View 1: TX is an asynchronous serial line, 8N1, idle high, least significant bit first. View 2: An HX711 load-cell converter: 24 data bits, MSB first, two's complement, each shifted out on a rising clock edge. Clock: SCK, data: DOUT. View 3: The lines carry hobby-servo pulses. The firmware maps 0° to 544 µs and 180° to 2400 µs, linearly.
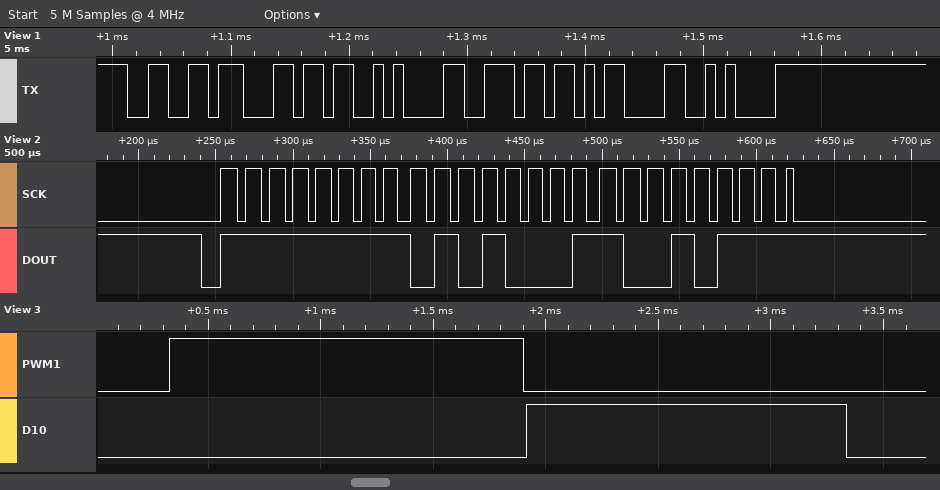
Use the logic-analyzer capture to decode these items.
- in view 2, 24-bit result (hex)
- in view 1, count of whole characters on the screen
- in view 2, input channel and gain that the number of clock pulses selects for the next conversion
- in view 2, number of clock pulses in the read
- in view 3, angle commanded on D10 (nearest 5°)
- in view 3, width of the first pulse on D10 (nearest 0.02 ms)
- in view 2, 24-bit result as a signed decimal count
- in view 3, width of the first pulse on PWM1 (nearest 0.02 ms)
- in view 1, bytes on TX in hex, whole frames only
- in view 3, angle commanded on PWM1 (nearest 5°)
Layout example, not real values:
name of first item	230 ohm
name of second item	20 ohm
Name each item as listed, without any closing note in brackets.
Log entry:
in view 2, 24-bit result	0xFF5197
in view 1, count of whole characters on the screen	6
in view 2, input channel and gain that the number of clock pulses selects for the next conversion	channel A, gain 128
in view 2, number of clock pulses in the read	25
in view 3, angle commanded on D10	85°
in view 3, width of the first pulse on D10	1.42 ms
in view 2, 24-bit result as a signed decimal count	-44649
in view 3, width of the first pulse on PWM1	1.58 ms
in view 1, bytes on TX in hex, whole frames only	66 6C 0A 6E 0D 0A
in view 3, angle commanded on PWM1	100°
